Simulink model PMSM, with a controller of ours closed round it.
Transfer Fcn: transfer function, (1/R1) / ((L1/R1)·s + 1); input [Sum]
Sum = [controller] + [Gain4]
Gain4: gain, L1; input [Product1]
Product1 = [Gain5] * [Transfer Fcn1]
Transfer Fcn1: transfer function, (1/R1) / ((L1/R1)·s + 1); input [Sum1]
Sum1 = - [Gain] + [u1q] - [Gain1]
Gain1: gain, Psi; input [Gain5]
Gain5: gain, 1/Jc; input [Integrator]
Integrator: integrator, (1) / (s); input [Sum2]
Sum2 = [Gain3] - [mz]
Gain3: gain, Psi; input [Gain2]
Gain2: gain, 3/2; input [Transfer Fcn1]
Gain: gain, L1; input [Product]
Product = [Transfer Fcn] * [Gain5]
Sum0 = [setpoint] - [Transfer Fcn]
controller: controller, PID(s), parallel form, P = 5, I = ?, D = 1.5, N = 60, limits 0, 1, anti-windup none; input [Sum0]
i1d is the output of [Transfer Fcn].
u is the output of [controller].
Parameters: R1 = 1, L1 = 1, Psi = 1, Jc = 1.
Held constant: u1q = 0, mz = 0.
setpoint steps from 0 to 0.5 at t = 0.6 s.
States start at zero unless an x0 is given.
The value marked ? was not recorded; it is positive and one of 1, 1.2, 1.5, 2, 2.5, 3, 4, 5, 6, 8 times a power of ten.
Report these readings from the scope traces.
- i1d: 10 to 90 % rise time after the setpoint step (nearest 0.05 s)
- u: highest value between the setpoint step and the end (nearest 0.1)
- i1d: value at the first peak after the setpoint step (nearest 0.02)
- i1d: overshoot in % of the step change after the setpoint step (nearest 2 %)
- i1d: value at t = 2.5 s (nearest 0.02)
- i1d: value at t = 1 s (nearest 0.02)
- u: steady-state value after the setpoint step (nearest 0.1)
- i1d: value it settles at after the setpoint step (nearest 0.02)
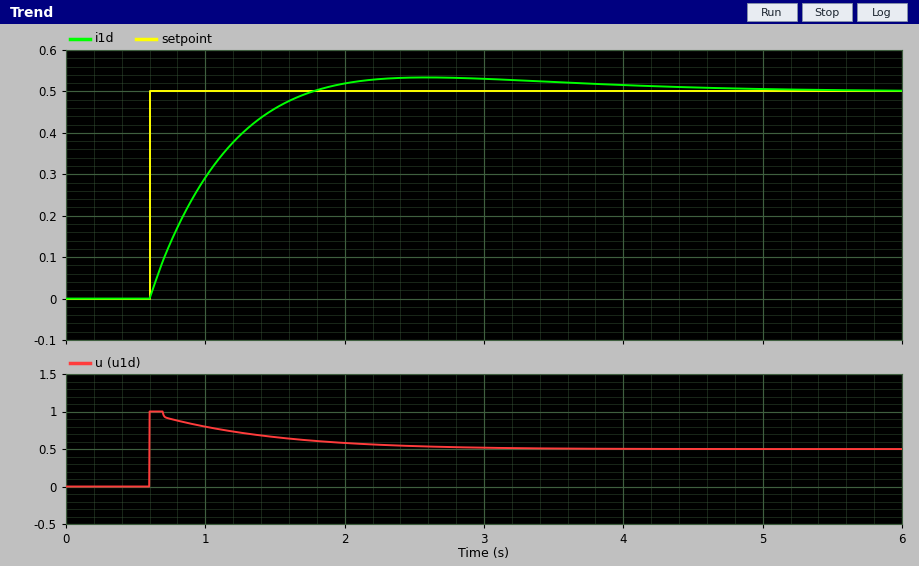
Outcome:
0.80 s
1.0
0.54
6 %
0.54
0.30
0.5
0.50
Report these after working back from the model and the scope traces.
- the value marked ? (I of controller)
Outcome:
4
